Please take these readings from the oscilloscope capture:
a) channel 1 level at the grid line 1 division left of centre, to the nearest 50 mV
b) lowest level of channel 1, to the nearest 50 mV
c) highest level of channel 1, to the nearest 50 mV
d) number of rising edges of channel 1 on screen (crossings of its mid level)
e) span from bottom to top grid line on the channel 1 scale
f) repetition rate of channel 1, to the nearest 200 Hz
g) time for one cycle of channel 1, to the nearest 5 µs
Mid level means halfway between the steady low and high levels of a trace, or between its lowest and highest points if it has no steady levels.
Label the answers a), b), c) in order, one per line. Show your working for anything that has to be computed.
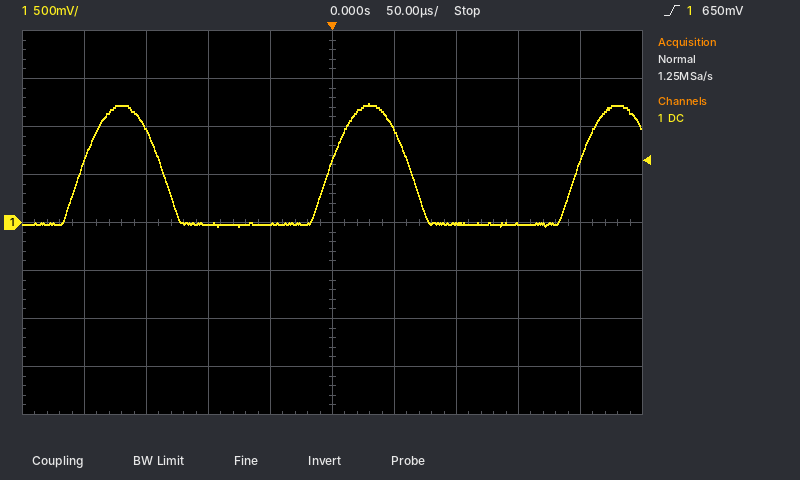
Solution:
a) 0 mV
b) -50 mV
c) 1.25 V
d) 3
e) 4 V
f) 1 / 200 µs ≈ 5.0 kHz
g) 200 µs
